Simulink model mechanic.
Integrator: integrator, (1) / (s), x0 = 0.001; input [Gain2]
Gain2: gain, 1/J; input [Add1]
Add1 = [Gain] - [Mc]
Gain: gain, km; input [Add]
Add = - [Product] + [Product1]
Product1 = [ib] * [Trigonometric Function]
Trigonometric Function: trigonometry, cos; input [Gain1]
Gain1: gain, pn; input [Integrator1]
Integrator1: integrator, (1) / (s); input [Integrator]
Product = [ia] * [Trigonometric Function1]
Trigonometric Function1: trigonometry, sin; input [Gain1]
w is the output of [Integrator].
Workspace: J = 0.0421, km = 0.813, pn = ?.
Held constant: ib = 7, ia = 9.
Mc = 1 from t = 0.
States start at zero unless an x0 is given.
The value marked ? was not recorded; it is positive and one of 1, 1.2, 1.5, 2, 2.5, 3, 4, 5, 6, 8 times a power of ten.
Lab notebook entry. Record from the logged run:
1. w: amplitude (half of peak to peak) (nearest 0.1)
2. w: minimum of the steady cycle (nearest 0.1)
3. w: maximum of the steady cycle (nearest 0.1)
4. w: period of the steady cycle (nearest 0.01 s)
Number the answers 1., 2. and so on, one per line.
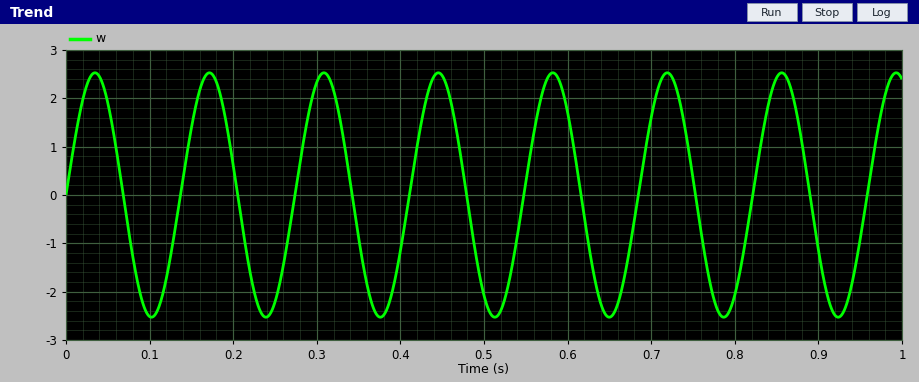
1. 2.5
2. -2.5
3. 2.5
4. 0.14 s
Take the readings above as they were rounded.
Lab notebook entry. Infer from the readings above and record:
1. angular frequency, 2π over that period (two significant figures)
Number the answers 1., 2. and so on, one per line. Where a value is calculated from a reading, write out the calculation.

1. 2π / 0.14 = 45 rad/s
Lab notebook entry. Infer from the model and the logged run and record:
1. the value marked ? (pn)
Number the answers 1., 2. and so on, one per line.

1. 10
